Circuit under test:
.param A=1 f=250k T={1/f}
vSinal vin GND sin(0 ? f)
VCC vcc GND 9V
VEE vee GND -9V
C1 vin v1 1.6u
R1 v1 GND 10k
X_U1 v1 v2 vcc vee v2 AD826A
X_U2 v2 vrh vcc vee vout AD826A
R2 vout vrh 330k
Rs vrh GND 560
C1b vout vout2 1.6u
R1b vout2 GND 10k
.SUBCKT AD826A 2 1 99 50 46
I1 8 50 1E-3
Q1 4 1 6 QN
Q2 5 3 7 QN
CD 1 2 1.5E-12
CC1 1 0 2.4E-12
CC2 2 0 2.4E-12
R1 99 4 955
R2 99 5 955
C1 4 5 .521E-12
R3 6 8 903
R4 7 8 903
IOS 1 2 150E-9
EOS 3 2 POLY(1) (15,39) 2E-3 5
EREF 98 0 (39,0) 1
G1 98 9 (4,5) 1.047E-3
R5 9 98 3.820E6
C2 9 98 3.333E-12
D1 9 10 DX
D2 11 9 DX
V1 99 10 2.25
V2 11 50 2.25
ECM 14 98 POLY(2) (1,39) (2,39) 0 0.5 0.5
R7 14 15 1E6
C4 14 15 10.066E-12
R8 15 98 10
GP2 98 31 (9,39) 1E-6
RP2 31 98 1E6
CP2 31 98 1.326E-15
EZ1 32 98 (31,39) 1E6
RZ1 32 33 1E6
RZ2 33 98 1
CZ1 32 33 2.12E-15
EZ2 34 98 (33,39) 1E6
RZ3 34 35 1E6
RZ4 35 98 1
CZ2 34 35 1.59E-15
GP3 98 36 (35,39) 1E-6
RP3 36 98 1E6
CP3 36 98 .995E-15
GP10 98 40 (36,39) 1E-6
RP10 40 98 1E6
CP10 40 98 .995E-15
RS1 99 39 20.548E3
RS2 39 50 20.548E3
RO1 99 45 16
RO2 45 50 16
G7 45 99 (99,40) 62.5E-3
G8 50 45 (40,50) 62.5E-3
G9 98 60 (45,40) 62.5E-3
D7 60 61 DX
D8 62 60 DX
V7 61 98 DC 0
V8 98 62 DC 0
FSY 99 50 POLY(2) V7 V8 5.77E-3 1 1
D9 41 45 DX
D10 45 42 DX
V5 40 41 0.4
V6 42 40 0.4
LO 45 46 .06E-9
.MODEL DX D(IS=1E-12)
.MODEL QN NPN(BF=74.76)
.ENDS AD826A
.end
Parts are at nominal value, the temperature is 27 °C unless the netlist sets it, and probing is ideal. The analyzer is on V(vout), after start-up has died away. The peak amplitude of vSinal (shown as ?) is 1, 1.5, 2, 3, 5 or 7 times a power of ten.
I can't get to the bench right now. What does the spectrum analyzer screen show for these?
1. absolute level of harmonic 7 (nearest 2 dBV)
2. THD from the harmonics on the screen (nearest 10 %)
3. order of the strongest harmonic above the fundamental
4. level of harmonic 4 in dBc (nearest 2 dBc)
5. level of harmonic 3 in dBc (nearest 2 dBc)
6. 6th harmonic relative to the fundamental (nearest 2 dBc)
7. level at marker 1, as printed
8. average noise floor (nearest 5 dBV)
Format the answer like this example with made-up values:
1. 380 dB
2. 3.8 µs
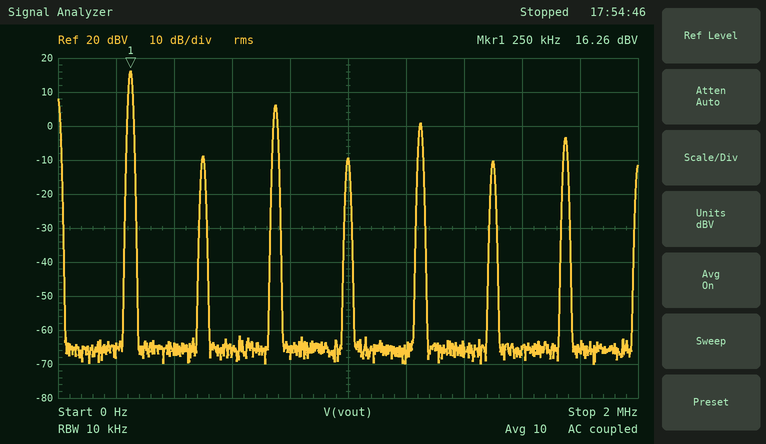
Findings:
1. -4 dBV
2. 40 %
3. 3
4. -26 dBc
5. -10 dBc
6. -26 dBc
7. 16.26 dBV
8. -65 dBV
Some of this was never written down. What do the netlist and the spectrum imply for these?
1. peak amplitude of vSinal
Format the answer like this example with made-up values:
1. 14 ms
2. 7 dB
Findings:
1. 1 V
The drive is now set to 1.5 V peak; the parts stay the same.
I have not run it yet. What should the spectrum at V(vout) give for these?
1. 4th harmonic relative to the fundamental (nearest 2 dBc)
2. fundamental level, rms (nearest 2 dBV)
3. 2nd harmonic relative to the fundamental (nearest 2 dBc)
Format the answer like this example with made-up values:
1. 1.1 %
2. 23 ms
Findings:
1. -28 dBc
2. 16 dBV
3. -28 dBc
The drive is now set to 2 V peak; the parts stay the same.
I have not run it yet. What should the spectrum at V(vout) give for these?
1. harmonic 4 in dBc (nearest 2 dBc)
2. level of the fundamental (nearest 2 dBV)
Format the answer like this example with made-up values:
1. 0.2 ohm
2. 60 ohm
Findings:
1. -32 dBc
2. 16 dBV
